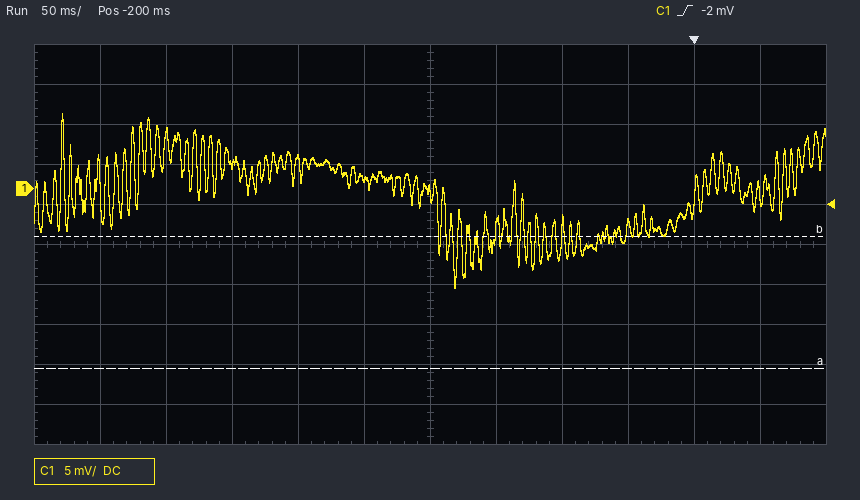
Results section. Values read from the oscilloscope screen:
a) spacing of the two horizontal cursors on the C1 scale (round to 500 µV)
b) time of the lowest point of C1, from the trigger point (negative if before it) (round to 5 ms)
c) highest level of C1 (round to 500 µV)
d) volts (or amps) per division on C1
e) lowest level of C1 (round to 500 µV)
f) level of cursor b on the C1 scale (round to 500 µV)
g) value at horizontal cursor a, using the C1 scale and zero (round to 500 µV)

16.5 mV
-180 ms
9.5 mV
5 mV
-12.5 mV
-6.0 mV
-22.5 mV
